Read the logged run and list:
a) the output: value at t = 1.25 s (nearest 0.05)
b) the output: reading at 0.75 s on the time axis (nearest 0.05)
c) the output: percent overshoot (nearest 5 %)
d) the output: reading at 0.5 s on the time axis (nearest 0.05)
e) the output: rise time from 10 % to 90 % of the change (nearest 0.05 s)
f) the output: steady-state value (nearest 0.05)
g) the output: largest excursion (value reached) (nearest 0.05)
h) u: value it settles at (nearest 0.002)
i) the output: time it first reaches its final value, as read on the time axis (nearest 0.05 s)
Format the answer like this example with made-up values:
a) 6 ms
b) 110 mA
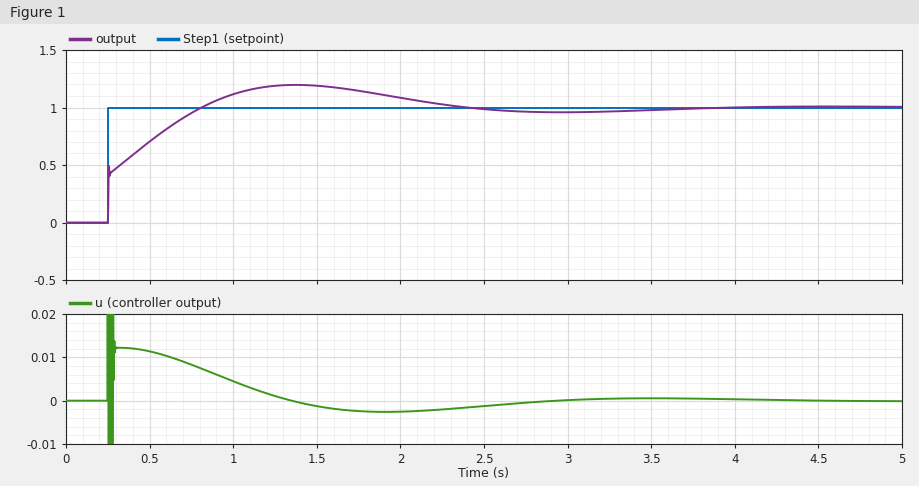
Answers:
a) 1.20
b) 0.95
c) 20 %
d) 0.70
e) 0.45 s
f) 1.00
g) 1.20
h) 0.000
i) 0.80 s
